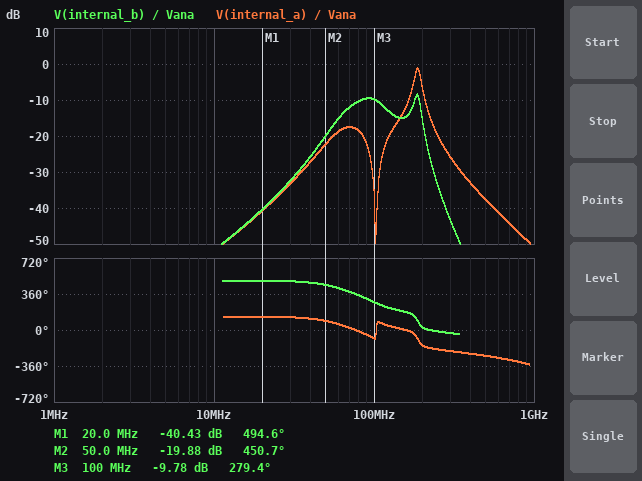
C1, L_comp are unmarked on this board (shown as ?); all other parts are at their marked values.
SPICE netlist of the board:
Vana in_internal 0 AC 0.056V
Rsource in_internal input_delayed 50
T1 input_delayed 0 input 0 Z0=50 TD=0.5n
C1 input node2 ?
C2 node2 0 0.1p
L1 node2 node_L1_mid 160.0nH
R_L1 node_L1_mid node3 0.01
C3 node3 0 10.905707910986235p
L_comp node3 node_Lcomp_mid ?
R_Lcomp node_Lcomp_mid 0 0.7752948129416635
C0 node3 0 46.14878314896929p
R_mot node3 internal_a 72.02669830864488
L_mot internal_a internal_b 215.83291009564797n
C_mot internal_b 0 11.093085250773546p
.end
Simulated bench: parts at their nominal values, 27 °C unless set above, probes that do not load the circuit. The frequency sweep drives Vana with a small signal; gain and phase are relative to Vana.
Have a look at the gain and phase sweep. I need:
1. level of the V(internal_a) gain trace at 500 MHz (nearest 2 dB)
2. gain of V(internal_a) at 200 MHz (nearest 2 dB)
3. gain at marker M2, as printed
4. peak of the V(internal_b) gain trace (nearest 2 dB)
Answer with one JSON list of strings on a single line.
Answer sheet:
["-38 dB", "-6 dB", "-19.88 dB", "-8 dB"]
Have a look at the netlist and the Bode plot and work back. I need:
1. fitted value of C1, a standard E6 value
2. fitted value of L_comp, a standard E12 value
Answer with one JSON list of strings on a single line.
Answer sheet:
["33 pF", "15 nH"]
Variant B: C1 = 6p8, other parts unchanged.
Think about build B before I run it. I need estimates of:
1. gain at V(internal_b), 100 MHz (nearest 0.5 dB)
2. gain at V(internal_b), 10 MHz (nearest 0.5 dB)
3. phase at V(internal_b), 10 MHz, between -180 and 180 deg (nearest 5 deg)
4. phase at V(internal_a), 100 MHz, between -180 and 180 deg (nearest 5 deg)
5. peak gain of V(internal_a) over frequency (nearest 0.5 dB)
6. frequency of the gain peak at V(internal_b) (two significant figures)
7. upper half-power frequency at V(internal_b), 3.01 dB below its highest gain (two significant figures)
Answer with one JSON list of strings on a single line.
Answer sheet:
["-13.5 dB", "-65.5 dB", "135 deg", "35 deg", "0 dB", "140 MHz", "200 MHz"]
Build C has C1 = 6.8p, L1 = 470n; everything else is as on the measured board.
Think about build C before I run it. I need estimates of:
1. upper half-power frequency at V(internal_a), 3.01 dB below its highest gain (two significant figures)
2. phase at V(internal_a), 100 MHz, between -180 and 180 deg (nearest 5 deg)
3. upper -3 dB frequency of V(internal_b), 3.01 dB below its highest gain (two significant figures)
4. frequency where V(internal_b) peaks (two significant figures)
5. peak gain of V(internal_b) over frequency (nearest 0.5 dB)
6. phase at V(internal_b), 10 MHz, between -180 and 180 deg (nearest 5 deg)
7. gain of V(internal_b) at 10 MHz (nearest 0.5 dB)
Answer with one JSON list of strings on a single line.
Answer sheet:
["190 MHz", "-85 deg", "99 MHz", "88 MHz", "-7.5 dB", "135 deg", "-65.5 dB"]
